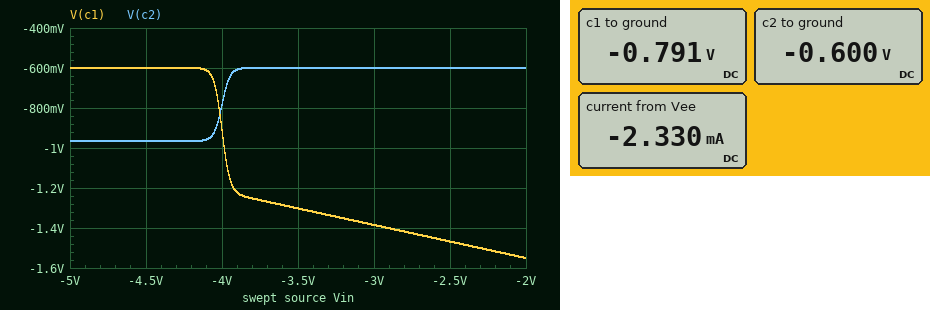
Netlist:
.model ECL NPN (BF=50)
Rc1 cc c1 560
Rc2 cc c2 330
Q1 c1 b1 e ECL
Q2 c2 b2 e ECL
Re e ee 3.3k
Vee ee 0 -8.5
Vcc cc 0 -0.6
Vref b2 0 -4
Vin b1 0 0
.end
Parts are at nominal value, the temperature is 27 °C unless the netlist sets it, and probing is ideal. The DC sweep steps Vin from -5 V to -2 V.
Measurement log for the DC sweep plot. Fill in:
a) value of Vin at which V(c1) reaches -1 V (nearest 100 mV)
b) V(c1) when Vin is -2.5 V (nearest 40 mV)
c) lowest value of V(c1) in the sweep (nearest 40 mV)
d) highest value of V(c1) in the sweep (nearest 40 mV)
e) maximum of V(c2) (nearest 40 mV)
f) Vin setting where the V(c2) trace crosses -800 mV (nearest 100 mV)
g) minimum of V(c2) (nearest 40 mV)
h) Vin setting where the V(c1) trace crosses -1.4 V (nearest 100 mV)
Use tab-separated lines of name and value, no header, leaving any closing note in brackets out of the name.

value of Vin at which V(c1) reaches -1 V	-4.0 V
V(c1) when Vin is -2.5 V	-1.48 V
lowest value of V(c1) in the sweep	-1.56 V
highest value of V(c1) in the sweep	-600 mV
maximum of V(c2)	-600 mV
Vin setting where the V(c2) trace crosses -800 mV	-4.0 V
minimum of V(c2)	-960 mV
Vin setting where the V(c1) trace crosses -1.4 V	-2.9 V
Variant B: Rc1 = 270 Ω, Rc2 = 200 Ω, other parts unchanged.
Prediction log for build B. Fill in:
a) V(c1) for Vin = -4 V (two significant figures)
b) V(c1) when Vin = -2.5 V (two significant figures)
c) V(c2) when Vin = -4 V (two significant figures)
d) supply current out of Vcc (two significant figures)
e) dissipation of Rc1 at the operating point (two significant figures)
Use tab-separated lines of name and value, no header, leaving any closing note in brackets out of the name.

V(c1) for Vin = -4 V	-750 mV
V(c1) when Vin = -2.5 V	-1.0 V
V(c2) when Vin = -4 V	-710 mV
supply current out of Vcc	690 µA
dissipation of Rc1 at the operating point	130 µW
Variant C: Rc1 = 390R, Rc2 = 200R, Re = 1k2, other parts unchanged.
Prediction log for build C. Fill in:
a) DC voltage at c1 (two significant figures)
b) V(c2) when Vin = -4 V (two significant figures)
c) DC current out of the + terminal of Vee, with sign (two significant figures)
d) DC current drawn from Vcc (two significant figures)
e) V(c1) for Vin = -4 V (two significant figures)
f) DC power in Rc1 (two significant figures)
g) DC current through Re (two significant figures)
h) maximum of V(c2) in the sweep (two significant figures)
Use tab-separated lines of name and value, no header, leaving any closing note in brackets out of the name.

DC voltage at c1	-820 mV
V(c2) when Vin = -4 V	-900 mV
DC current out of the + terminal of Vee, with sign	-6.4 mA
DC current drawn from Vcc	560 µA
V(c1) for Vin = -4 V	-1.2 V
DC power in Rc1	120 µW
DC current through Re	6.4 mA
maximum of V(c2) in the sweep	-600 mV
